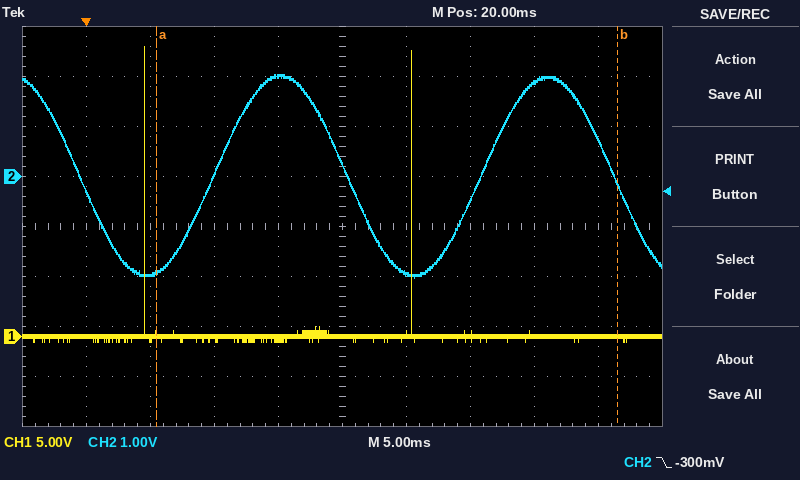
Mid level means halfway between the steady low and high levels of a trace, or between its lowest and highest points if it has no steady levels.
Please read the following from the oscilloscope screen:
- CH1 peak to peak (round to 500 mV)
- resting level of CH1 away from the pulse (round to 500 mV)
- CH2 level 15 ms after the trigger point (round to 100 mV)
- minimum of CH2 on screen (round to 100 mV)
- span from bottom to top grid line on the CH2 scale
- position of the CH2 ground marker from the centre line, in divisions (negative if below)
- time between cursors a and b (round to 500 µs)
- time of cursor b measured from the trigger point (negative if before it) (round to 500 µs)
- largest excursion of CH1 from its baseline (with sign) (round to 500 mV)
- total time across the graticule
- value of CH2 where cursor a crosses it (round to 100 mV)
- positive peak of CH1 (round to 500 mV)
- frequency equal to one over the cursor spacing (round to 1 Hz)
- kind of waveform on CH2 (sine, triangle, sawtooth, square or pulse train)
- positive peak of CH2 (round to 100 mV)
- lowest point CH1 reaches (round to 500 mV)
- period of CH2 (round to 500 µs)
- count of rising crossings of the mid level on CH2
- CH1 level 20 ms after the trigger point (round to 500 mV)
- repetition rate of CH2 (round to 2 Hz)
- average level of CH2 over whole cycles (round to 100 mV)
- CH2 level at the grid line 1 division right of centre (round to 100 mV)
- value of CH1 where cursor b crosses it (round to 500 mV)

29.5 V
0.0 V
2.0 V
-2.0 V
8 V
+1.0 div
36.0 ms
+41.5 ms
+29.0 V
50 ms
-1.9 V
29.0 V
28 Hz
sine
2.0 V
-500 mV
21.0 ms
2
0.0 V
48 Hz
0.0 V
-1.9 V
0.0 V
